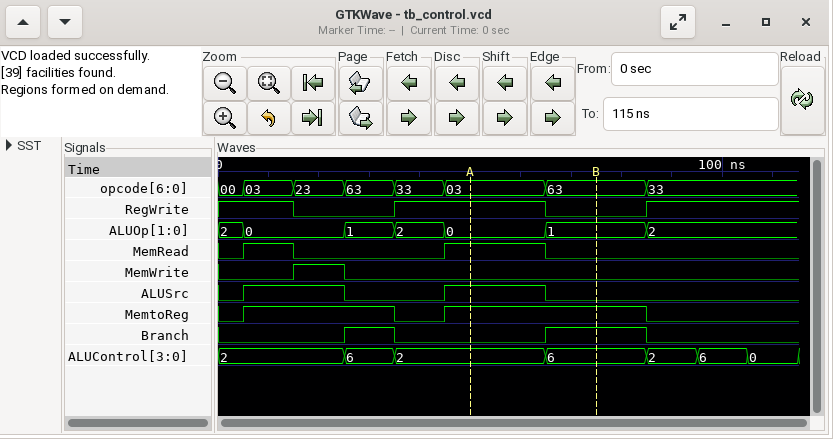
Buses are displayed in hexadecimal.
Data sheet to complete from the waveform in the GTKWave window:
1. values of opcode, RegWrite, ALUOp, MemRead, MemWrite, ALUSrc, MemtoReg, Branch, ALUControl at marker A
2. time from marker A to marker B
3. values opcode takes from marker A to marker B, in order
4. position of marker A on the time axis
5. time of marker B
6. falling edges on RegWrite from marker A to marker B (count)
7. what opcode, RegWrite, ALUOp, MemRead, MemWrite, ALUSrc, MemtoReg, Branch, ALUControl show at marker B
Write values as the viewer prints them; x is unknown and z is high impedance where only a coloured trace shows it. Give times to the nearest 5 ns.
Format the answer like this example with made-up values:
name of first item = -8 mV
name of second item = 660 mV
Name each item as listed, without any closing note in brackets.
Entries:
values of opcode, RegWrite, ALUOp, MemRead, MemWrite, ALUSrc, MemtoReg, Branch, ALUControl at marker A = opcode=03, RegWrite=1, ALUOp=0, MemRead=1, MemWrite=0, ALUSrc=1, MemtoReg=1, Branch=0, ALUControl=2
time from marker A to marker B = 25 ns
values opcode takes from marker A to marker B, in order = 03, 63
position of marker A on the time axis = 50 ns
time of marker B = 75 ns
falling edges on RegWrite from marker A to marker B = 1
what opcode, RegWrite, ALUOp, MemRead, MemWrite, ALUSrc, MemtoReg, Branch, ALUControl show at marker B = opcode=63, RegWrite=0, ALUOp=1, MemRead=0, MemWrite=0, ALUSrc=0, MemtoReg=1, Branch=1, ALUControl=6
